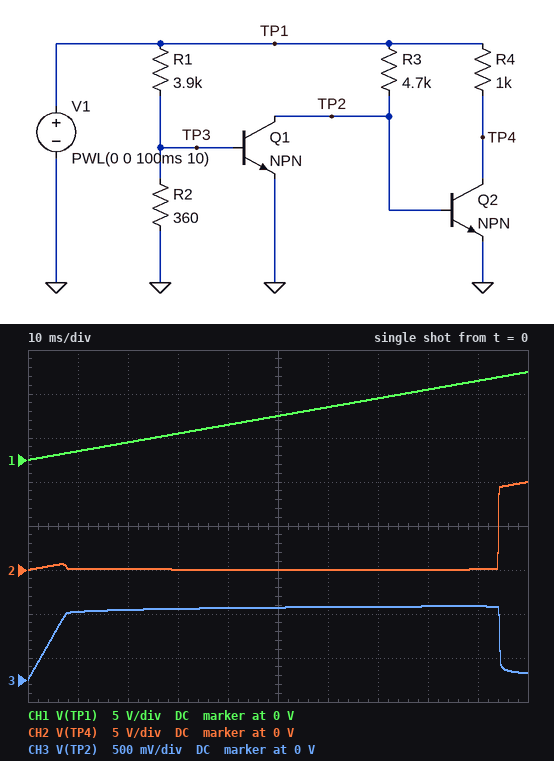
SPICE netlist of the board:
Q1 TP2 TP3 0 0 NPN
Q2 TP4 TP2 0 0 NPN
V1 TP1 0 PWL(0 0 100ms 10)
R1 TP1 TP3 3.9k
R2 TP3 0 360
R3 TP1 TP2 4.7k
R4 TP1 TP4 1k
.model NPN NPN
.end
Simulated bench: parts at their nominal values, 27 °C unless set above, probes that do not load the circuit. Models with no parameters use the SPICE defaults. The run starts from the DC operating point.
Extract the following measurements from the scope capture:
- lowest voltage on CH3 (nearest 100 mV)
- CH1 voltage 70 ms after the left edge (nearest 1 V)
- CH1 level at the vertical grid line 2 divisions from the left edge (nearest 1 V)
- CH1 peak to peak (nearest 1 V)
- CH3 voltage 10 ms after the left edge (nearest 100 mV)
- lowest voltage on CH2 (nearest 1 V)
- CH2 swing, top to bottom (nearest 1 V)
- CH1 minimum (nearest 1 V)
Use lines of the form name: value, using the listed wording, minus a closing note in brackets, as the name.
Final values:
lowest voltage on CH3: 0 V
CH1 voltage 70 ms after the left edge: 7 V
CH1 level at the vertical grid line 2 divisions from the left edge: 2 V
CH1 peak to peak: 10 V
CH3 voltage 10 ms after the left edge: 800 mV
lowest voltage on CH2: 0 V
CH2 swing, top to bottom: 10 V
CH1 minimum: 0 V
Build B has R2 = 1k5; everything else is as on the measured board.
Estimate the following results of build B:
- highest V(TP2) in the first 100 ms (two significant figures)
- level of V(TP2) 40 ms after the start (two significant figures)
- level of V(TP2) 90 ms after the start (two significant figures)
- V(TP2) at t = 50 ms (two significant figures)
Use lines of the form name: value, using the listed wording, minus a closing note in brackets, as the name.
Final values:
highest V(TP2) in the first 100 ms: 800 mV
level of V(TP2) 40 ms after the start: 41 mV
level of V(TP2) 90 ms after the start: 31 mV
V(TP2) at t = 50 ms: 36 mV
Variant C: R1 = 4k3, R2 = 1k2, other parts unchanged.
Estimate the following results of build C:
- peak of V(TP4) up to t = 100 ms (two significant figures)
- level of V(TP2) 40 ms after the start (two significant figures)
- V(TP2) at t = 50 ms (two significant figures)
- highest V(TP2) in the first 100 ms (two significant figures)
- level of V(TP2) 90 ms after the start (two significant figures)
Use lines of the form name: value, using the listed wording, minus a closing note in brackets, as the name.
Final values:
peak of V(TP4) up to t = 100 ms: 10 V
level of V(TP2) 40 ms after the start: 62 mV
V(TP2) at t = 50 ms: 44 mV
highest V(TP2) in the first 100 ms: 810 mV
level of V(TP2) 90 ms after the start: 33 mV
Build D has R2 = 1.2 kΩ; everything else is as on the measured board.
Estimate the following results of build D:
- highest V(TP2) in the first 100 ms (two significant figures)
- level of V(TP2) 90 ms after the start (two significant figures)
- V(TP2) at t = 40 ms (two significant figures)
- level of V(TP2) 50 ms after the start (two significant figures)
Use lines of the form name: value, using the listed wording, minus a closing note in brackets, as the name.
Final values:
highest V(TP2) in the first 100 ms: 810 mV
level of V(TP2) 90 ms after the start: 32 mV
V(TP2) at t = 40 ms: 51 mV
level of V(TP2) 50 ms after the start: 40 mV
